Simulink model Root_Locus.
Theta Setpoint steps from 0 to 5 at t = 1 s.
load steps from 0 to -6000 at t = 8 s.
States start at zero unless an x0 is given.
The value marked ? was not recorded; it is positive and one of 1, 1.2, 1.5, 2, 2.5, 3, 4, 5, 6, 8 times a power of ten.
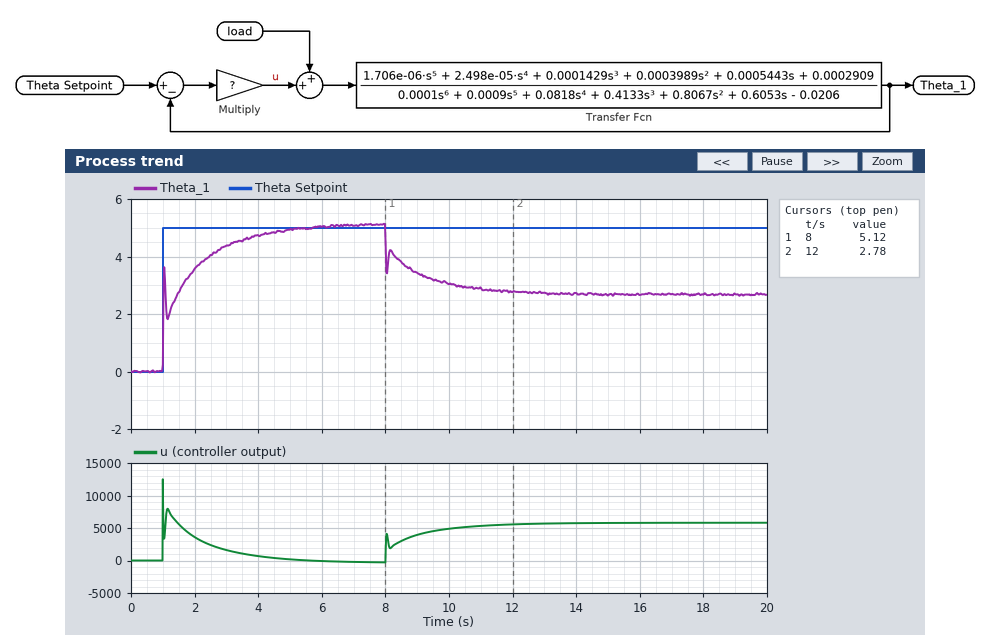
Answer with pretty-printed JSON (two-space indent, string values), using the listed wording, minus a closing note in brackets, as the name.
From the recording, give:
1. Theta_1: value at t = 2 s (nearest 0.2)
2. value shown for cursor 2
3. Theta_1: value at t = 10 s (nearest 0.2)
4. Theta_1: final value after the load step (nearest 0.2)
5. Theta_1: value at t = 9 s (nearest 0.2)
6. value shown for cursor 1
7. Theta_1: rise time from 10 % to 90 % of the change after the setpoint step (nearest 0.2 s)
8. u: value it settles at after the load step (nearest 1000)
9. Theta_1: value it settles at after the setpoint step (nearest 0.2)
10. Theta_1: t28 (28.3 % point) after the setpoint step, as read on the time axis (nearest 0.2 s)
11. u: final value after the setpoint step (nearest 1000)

{
  "Theta_1: value at t = 2 s": "3.6",
  "value shown for cursor 2": "2.78",
  "Theta_1: value at t = 10 s": "3.0",
  "Theta_1: final value after the load step": "2.6",
  "Theta_1: value at t = 9 s": "3.4",
  "value shown for cursor 1": "5.12",
  "Theta_1: rise time from 10 % to 90 % of the change after the setpoint step": "2.6 s",
  "u: value it settles at after the load step": "6000",
  "Theta_1: value it settles at after the setpoint step": "5.2",
  "Theta_1: t28 (28.3 % point) after the setpoint step, as read on the time axis": "1.0 s",
  "u: final value after the setpoint step": "0"
}
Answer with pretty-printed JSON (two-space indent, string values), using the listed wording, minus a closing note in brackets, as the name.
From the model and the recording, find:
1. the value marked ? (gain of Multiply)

{
  "the value marked ?": "2500"
}
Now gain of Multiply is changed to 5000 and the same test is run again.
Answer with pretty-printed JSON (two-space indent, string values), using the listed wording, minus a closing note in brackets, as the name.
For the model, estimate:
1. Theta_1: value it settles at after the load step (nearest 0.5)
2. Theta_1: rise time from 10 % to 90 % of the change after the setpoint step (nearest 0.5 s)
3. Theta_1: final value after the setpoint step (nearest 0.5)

{
  "Theta_1: value it settles at after the load step": "4.0",
  "Theta_1: rise time from 10 % to 90 % of the change after the setpoint step": "1.5 s",
  "Theta_1: final value after the setpoint step": "5.0"
}
